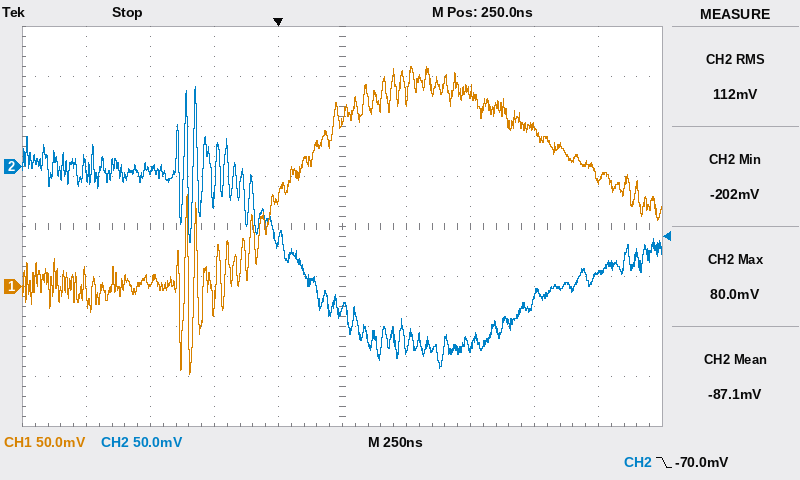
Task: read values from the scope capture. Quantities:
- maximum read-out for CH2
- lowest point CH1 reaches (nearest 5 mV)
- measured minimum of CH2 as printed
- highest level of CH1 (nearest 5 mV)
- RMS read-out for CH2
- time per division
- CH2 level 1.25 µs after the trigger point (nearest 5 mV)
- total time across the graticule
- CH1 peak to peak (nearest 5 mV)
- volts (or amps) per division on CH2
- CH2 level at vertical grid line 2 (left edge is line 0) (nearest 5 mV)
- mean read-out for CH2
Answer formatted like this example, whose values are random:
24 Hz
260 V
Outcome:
80.0 mV
-90 mV
-202 mV
220 mV
112 mV
250 ns
-105 mV
2.5 µs
310 mV
50 mV
-5 mV
-87.1 mV
